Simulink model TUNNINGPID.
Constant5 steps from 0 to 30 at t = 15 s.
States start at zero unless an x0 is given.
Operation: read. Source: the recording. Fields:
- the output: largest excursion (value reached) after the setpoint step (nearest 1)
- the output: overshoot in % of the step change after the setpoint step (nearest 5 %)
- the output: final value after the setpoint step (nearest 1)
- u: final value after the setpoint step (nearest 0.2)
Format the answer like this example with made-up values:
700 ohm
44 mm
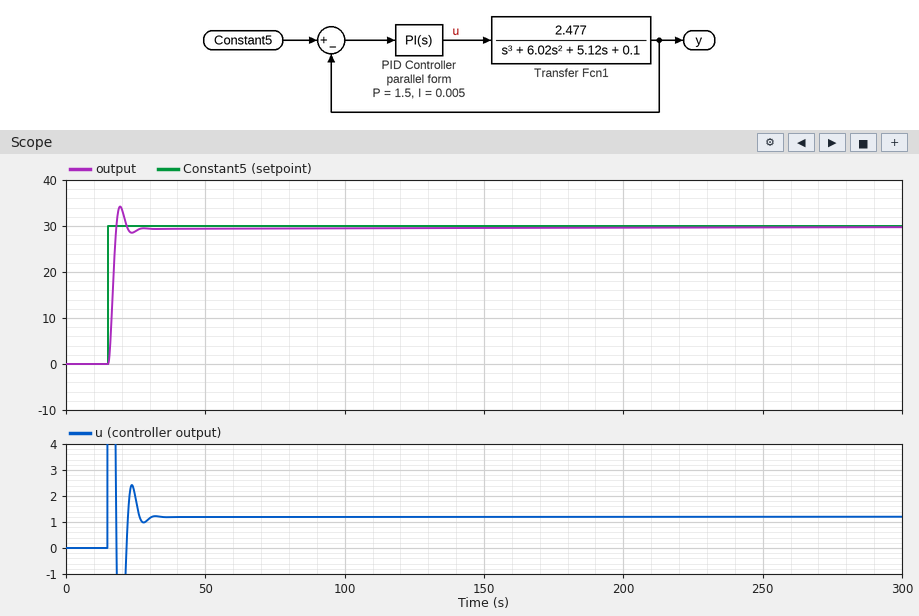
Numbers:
34
15 %
30
1.2
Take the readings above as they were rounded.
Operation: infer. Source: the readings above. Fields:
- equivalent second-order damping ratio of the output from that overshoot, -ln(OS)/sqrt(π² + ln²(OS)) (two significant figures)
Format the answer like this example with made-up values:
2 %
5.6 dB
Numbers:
0.52
